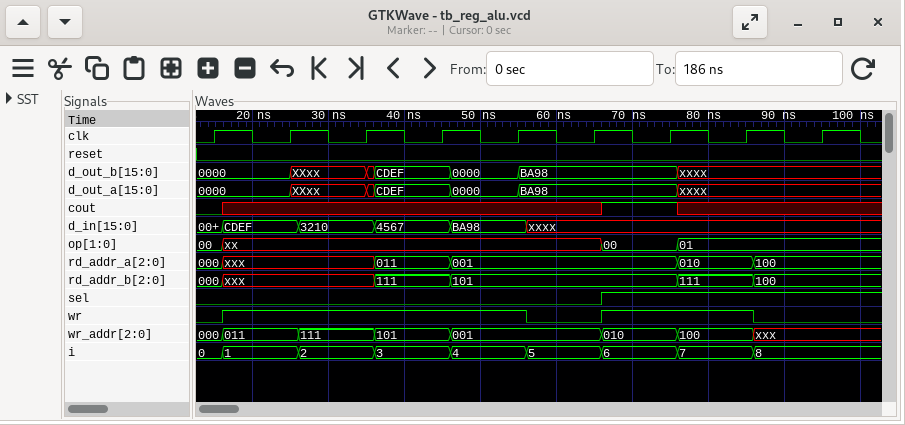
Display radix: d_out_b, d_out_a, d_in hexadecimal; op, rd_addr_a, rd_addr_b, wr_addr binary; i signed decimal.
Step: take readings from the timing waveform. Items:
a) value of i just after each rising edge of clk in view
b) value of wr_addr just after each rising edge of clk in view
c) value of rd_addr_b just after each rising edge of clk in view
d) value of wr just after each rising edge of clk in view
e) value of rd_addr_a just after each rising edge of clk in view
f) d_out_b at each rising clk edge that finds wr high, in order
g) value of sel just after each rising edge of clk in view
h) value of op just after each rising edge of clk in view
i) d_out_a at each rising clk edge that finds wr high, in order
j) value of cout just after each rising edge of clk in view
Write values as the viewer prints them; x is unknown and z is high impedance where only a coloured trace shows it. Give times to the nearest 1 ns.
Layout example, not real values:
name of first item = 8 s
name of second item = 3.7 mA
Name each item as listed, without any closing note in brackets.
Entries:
value of i just after each rising edge of clk in view = 0, 1, 2, 3, 4, 5, 6, 7, 8
value of wr_addr just after each rising edge of clk in view = 000, 011, 111, 101, 001, 001, 010, 100, xxx
value of rd_addr_b just after each rising edge of clk in view = 000, xxx, xxx, 111, 101, 101, 101, 111, 100
value of wr just after each rising edge of clk in view = 0 1 1 1 1 0 1 1 0
value of rd_addr_a just after each rising edge of clk in view = 000, xxx, xxx, 011, 001, 001, 001, 010, 100
d_out_b at each rising clk edge that finds wr high, in order = 0000, XXxx, CDEF, 0000, BA98, xxxx
value of sel just after each rising edge of clk in view = 0 0 0 0 0 0 1 1 1
value of op just after each rising edge of clk in view = 00, xx, xx, xx, xx, xx, 00, 01, 01
d_out_a at each rising clk edge that finds wr high, in order = 0000, XXxx, CDEF, 0000, BA98, xxxx
value of cout just after each rising edge of clk in view = 0 x x x x x 1 x x
